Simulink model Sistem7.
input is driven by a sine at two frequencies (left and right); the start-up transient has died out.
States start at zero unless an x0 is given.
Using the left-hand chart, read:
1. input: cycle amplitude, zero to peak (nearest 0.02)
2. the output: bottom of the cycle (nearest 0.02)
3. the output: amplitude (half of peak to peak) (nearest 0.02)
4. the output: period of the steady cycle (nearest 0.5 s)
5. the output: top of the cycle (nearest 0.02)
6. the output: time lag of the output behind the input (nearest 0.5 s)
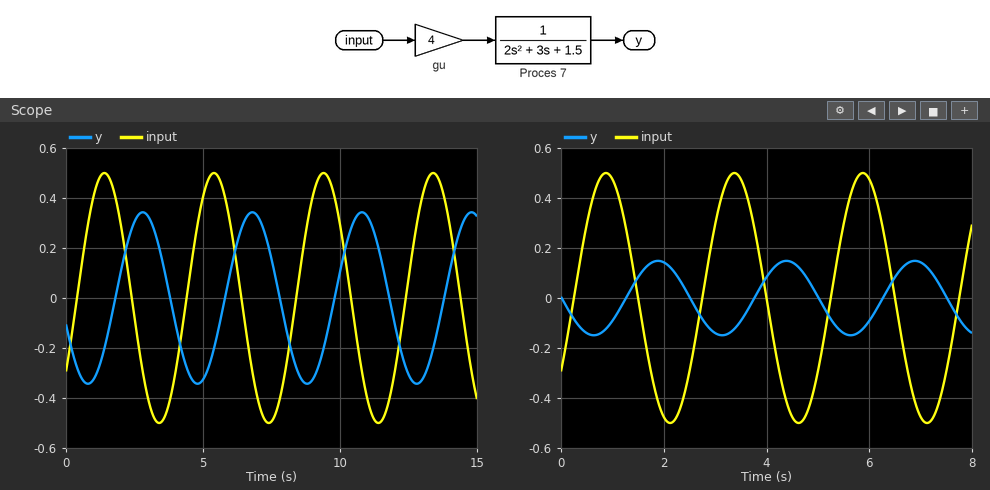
0.50
-0.34
0.34
4.0 s
0.34
1.5 s
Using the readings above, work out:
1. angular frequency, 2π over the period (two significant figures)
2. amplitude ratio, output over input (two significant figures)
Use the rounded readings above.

1.6 rad/s
0.68
